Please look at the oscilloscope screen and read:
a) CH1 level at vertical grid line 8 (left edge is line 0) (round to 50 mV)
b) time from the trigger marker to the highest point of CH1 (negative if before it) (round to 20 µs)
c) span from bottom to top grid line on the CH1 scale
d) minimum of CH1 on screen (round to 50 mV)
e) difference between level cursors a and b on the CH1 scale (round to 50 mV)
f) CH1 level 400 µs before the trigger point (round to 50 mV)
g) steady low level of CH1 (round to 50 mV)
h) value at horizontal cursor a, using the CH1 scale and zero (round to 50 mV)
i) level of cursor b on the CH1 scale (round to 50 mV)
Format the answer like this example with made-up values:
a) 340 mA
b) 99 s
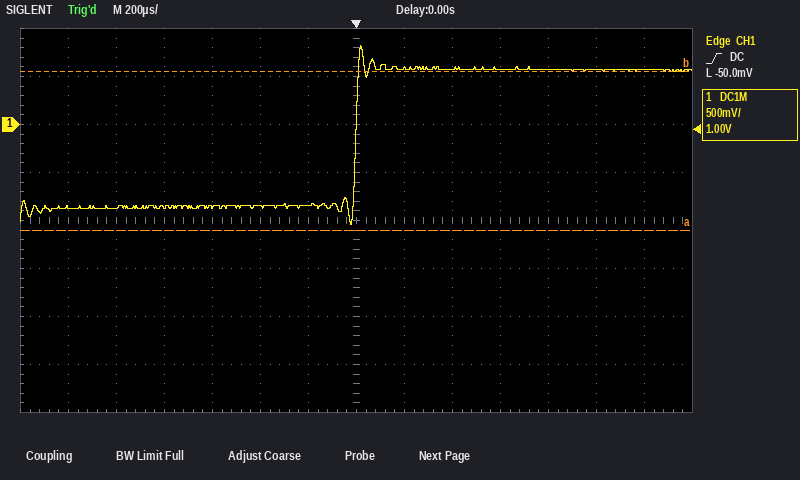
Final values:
a) 600 mV
b) +20 µs
c) 4 V
d) -1.05 V
e) 1.65 V
f) -850 mV
g) -850 mV
h) -1.10 V
i) 550 mV
